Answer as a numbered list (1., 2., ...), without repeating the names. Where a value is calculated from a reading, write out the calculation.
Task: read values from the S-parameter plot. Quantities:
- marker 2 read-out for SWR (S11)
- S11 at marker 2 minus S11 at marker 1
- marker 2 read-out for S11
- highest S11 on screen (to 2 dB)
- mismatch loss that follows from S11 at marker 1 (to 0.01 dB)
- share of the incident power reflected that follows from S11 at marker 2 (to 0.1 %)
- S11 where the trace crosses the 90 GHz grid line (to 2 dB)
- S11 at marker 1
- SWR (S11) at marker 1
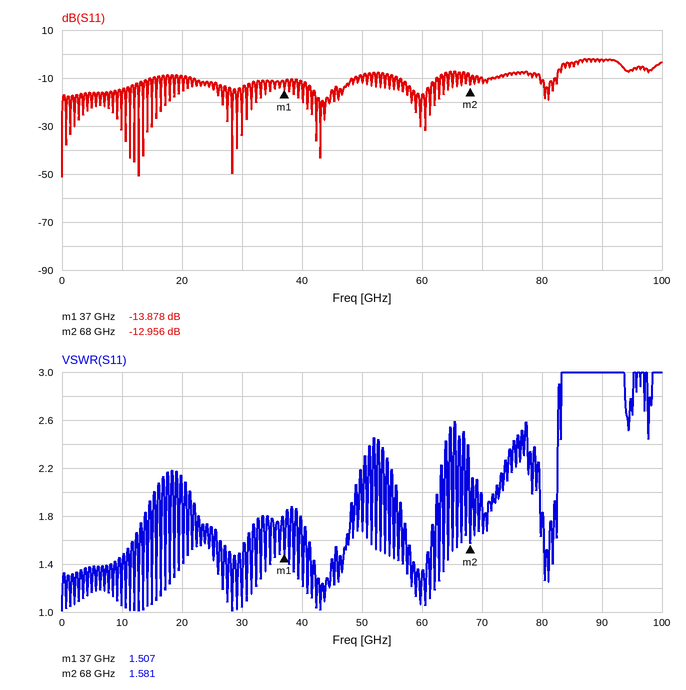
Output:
1. 1.581
2. -12.956 − (-13.878) = 0.922 dB
3. -12.956 dB
4. -2 dB
5. −10 log10(1 − 10^(-13.878/10)) ≈ 0.18 dB
6. 10^(-12.956/10) ≈ 5.1 %
7. -2 dB
8. -13.878 dB
9. 1.507
